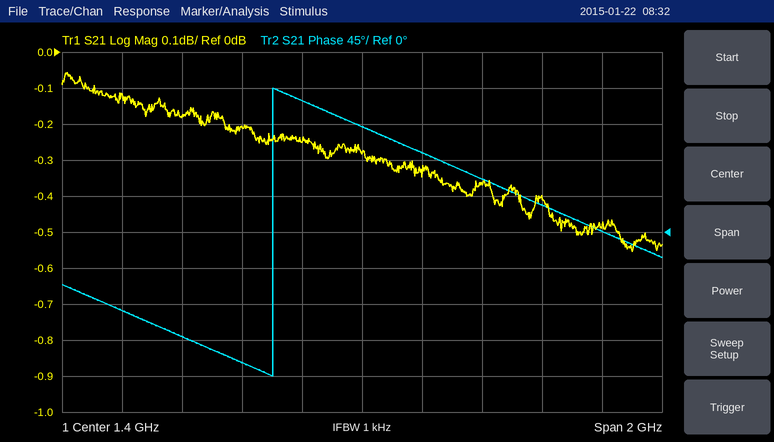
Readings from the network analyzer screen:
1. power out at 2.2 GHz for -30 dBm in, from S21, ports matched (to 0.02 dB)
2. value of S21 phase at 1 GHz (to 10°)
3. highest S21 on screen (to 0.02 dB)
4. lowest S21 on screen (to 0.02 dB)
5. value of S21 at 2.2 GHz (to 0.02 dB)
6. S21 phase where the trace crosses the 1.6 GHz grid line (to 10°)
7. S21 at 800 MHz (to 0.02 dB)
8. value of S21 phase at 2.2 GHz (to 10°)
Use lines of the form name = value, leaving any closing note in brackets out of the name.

power out at 2.2 GHz for -30 dBm in, from S21, ports matched = -30.48 dBm
value of S21 phase at 1 GHz = -160°
highest S21 on screen = -0.06 dB
lowest S21 on screen = -0.56 dB
value of S21 at 2.2 GHz = -0.48 dB
S21 phase where the trace crosses the 1.6 GHz grid line = 100°
S21 at 800 MHz = -0.18 dB
value of S21 phase at 2.2 GHz = 0°
